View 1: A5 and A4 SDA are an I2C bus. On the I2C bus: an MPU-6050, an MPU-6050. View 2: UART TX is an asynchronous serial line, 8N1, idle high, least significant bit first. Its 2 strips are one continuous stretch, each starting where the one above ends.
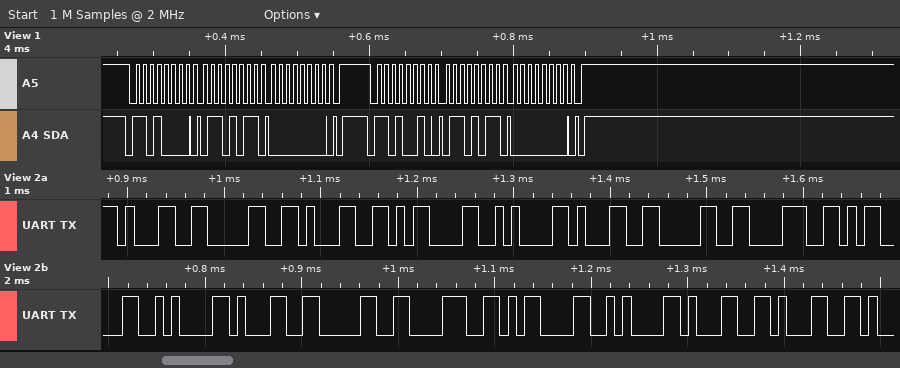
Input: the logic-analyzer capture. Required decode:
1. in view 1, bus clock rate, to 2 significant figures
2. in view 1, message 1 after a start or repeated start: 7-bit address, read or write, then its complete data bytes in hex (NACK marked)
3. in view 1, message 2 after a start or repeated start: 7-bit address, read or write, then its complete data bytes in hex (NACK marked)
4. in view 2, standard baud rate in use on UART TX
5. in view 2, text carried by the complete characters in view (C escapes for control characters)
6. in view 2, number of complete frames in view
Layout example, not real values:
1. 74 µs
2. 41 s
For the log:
1. 100 kHz
2. 0x68 write: 6B 00
3. 0x69 write: 6B 00
4. 115200 baud
5. "101\r\n108\r\n108\r\n11"
6. 17
